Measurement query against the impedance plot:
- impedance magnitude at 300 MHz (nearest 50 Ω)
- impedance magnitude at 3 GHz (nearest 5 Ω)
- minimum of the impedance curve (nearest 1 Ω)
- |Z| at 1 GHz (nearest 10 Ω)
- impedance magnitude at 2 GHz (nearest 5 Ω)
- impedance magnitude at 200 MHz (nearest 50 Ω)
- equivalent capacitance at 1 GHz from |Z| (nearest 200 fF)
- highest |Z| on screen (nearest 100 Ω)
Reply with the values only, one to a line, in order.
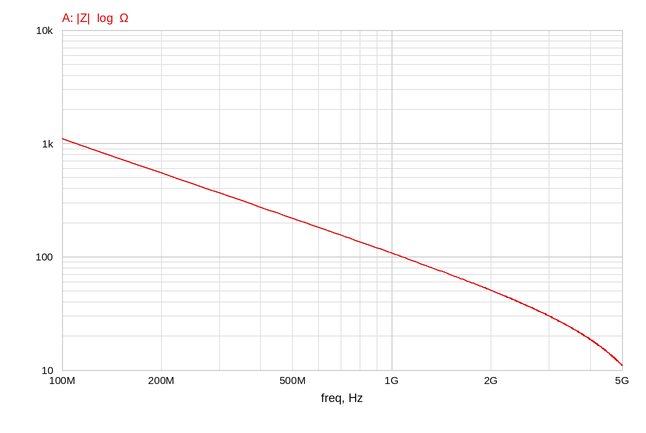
350 Ω
30 Ω
11 Ω
110 Ω
50 Ω
550 Ω
1.4 pF
1.1 kΩ
